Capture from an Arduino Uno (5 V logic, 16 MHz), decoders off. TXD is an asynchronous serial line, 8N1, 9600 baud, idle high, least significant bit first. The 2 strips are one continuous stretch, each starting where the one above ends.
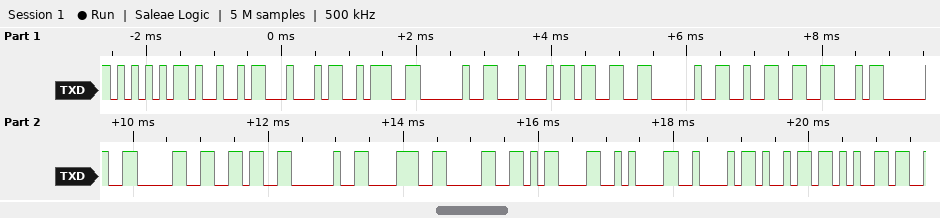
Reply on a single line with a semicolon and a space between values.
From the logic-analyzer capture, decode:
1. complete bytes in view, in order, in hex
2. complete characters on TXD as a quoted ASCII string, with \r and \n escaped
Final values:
55 49 44 3A 20 44 33 20 32 46 20 30 36 20 38 30 0D 0A 42 69 65; "UID: D3 2F 06 80\r\nBie"
